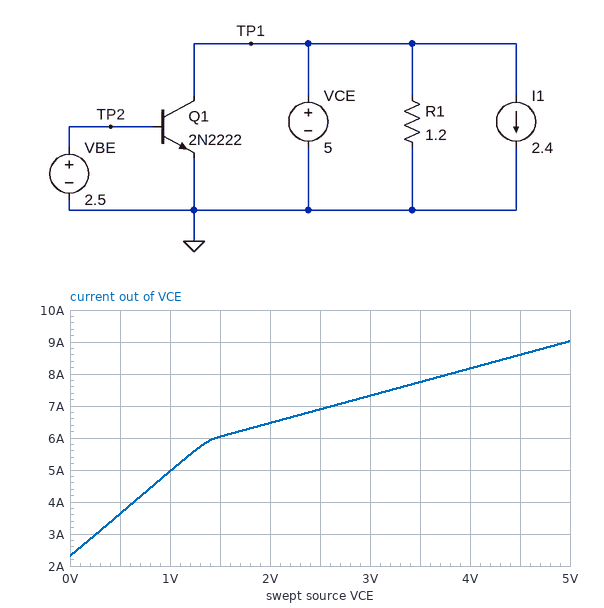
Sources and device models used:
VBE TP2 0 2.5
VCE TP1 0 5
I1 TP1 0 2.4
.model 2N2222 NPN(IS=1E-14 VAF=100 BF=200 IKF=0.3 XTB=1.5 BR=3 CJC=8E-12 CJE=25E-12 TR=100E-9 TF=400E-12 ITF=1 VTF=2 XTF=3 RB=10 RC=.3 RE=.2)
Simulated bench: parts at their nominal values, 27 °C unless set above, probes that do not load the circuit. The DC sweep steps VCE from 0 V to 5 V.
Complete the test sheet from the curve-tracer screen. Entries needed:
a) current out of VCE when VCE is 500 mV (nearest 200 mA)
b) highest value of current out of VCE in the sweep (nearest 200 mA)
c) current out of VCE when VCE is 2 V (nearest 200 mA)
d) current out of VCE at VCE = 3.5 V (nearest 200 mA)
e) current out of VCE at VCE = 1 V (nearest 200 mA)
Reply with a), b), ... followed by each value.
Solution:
a) 3.6 A
b) 9.0 A
c) 6.4 A
d) 7.8 A
e) 5.0 A
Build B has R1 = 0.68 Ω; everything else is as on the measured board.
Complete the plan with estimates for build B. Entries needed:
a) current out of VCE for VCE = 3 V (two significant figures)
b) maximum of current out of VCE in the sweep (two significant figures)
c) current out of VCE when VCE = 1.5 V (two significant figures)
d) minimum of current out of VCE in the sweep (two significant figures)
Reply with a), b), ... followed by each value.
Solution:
a) 9.2 A
b) 12 A
c) 7.0 A
d) 2.3 A
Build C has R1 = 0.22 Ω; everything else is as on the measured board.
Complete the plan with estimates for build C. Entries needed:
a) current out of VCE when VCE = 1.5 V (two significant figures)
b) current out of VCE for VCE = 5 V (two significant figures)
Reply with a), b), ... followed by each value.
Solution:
a) 12 A
b) 28 A
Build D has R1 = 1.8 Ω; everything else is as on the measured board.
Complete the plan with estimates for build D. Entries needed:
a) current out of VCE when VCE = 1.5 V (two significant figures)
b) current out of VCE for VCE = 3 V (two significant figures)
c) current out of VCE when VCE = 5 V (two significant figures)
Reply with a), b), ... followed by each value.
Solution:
a) 5.6 A
b) 6.5 A
c) 7.6 A
